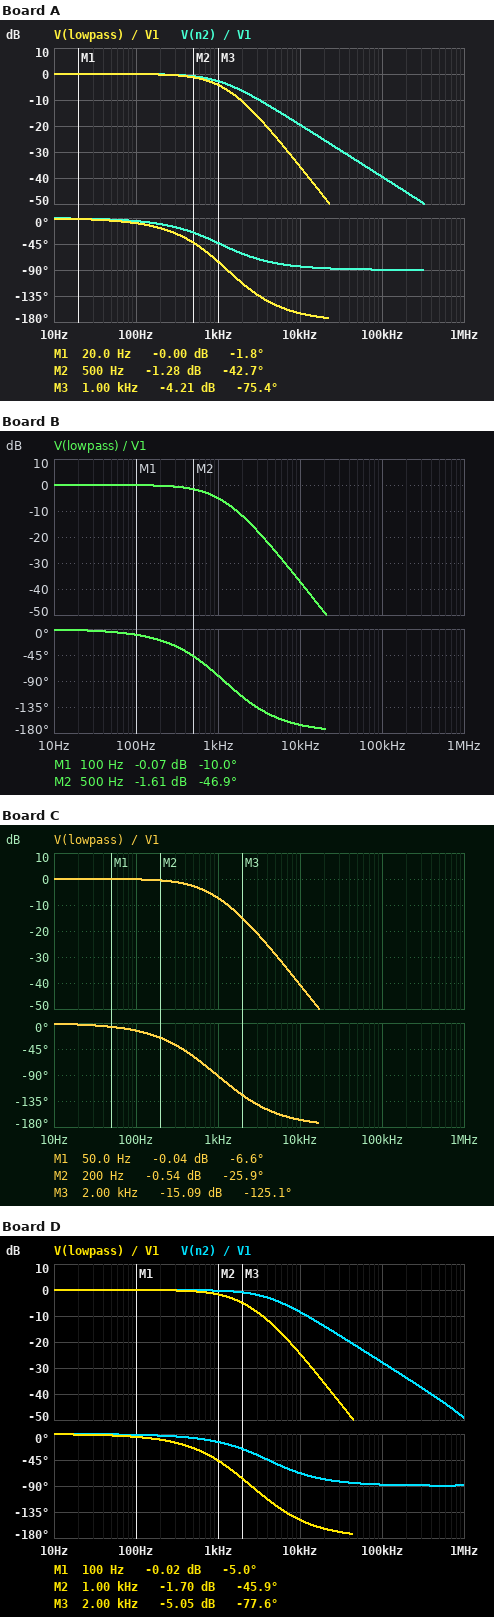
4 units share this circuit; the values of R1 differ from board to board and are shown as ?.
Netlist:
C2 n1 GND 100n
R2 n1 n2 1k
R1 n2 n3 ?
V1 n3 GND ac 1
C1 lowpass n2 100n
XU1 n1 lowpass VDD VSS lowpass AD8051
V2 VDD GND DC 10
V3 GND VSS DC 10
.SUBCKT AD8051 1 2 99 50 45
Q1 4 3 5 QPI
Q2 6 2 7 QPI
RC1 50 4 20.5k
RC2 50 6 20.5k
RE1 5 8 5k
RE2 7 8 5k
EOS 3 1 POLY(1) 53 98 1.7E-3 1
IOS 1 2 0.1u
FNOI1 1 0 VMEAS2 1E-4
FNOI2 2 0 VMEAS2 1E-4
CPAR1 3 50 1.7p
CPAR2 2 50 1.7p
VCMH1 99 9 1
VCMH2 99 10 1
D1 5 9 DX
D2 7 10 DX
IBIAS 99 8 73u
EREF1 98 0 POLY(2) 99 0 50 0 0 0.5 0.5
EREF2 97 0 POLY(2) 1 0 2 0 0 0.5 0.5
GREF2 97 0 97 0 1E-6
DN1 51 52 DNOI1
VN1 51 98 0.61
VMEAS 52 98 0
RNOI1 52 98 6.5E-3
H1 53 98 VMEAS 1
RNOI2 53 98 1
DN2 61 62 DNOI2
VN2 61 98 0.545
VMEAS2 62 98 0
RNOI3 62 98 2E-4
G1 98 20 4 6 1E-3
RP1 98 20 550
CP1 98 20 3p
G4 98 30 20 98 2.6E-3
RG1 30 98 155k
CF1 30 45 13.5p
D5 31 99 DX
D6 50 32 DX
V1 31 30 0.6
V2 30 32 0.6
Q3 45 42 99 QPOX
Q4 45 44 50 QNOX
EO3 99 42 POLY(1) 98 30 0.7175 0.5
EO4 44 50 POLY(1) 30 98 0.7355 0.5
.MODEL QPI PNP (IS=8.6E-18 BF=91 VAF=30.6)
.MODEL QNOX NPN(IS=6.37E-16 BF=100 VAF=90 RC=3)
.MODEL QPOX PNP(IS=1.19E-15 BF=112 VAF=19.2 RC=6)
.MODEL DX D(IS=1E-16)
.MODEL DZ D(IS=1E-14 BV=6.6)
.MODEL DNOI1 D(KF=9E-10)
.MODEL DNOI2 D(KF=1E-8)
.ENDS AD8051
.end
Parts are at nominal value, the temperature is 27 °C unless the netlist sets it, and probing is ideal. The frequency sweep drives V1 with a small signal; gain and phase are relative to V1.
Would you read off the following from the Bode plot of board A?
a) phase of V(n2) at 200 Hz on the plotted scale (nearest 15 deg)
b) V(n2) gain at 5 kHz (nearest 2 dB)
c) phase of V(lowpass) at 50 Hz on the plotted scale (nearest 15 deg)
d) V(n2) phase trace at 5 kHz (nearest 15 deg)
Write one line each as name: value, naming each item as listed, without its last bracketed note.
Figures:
phase of V(n2) at 200 Hz on the plotted scale: -15 deg
V(n2) gain at 5 kHz: -14 dB
phase of V(lowpass) at 50 Hz on the plotted scale: 0 deg
V(n2) phase trace at 5 kHz: -75 deg
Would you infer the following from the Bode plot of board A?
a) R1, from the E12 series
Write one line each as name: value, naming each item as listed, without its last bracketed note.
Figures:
R1, from the E12 series: 1.5 kΩ
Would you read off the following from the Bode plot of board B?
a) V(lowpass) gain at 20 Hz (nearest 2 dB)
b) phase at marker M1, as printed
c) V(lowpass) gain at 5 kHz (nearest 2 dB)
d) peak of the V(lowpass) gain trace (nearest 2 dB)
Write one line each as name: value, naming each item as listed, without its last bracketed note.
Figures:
V(lowpass) gain at 20 Hz: 0 dB
phase at marker M1, as printed: -10.0 deg
V(lowpass) gain at 5 kHz: -26 dB
peak of the V(lowpass) gain trace: 0 dB
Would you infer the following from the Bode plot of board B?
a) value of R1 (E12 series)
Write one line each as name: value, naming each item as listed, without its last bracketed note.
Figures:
value of R1: 1.8 kΩ
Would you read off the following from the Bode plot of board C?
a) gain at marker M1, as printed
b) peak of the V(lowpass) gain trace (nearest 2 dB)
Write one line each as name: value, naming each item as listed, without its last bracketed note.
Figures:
gain at marker M1, as printed: -0.04 dB
peak of the V(lowpass) gain trace: 0 dB
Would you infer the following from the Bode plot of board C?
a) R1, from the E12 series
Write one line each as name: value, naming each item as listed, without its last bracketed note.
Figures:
R1, from the E12 series: 2.7 kΩ
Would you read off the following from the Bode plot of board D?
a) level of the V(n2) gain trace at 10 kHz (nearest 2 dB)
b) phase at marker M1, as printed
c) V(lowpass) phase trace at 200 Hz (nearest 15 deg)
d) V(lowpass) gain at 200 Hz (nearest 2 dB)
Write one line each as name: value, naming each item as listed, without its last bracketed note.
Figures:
level of the V(n2) gain trace at 10 kHz: -8 dB
phase at marker M1, as printed: -5.0 deg
V(lowpass) phase trace at 200 Hz: -15 deg
V(lowpass) gain at 200 Hz: 0 dB
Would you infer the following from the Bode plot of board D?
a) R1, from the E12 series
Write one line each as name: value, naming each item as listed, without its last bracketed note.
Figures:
R1, from the E12 series: 390 Ω
